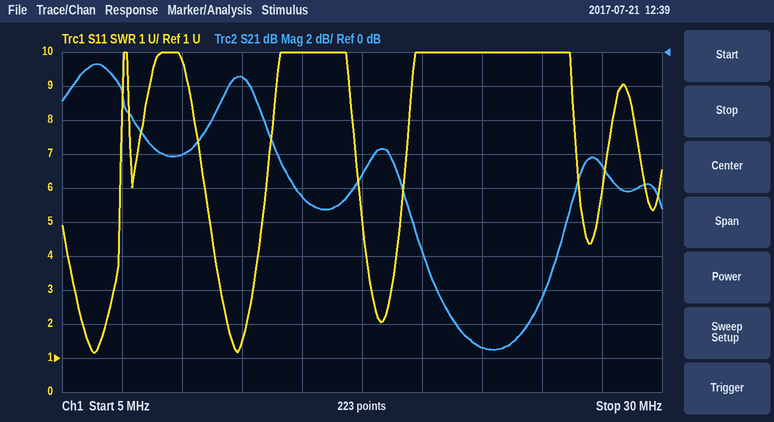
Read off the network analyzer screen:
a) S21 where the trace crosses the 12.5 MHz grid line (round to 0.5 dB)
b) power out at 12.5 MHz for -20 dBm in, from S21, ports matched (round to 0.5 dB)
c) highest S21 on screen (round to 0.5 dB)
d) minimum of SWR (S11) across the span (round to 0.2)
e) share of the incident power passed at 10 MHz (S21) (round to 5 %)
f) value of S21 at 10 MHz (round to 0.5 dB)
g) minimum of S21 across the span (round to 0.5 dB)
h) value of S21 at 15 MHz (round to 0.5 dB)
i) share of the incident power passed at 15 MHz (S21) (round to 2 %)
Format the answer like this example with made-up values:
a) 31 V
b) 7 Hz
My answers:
a) -1.5 dB
b) -21.5 dBm
c) -0.5 dB
d) 1.2
e) 25 %
f) -6.0 dB
g) -17.5 dB
h) -8.5 dB
i) 14 %
